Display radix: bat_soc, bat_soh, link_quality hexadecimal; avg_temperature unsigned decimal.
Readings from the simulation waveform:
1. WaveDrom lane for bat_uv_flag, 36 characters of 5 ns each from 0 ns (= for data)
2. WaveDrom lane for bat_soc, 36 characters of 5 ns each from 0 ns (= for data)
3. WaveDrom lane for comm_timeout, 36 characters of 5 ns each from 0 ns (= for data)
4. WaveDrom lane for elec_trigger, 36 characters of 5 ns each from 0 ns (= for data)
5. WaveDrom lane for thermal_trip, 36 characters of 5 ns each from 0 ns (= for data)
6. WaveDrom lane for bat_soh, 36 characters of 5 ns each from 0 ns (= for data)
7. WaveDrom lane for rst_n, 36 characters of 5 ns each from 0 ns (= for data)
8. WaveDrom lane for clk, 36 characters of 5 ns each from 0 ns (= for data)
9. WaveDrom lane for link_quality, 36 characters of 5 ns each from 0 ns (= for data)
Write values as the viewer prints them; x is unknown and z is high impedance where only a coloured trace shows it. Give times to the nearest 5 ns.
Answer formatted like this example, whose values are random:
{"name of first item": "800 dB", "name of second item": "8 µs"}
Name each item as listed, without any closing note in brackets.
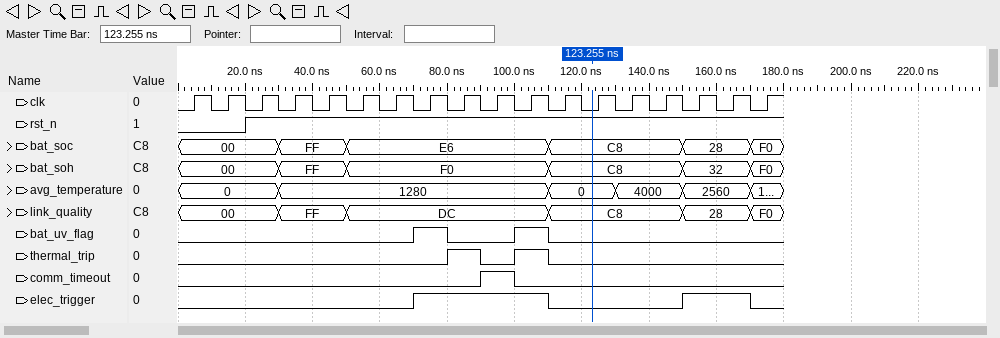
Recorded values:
{"WaveDrom lane for bat_uv_flag, 36 characters of 5 ns each from 0 ns": "{name: 'bat_uv_flag', wave: '0.............1.0...1.0.............'}", "WaveDrom lane for bat_soc, 36 characters of 5 ns each from 0 ns": "{name: 'bat_soc', wave: '=.....=...=...........=.......=...=.', data: '00 FF E6 C8 28 F0'}", "WaveDrom lane for comm_timeout, 36 characters of 5 ns each from 0 ns": "{name: 'comm_timeout', wave: '0.................1.0...............'}", "WaveDrom lane for elec_trigger, 36 characters of 5 ns each from 0 ns": "{name: 'elec_trigger', wave: '0.............1.......0.......1...0.'}", "WaveDrom lane for thermal_trip, 36 characters of 5 ns each from 0 ns": "{name: 'thermal_trip', wave: '0...............1.0.1.0.............'}", "WaveDrom lane for bat_soh, 36 characters of 5 ns each from 0 ns": "{name: 'bat_soh', wave: '=.....=...=...........=.......=...=.', data: '00 FF F0 C8 32 F0'}", "WaveDrom lane for rst_n, 36 characters of 5 ns each from 0 ns": "{name: 'rst_n', wave: '0...1...............................'}", "WaveDrom lane for clk, 36 characters of 5 ns each from 0 ns": "{name: 'clk', wave: '010101010101010101010101010101010101'}", "WaveDrom lane for link_quality, 36 characters of 5 ns each from 0 ns": "{name: 'link_quality', wave: '=.....=...=...........=.......=...=.', data: '00 FF DC C8 28 F0'}"}
